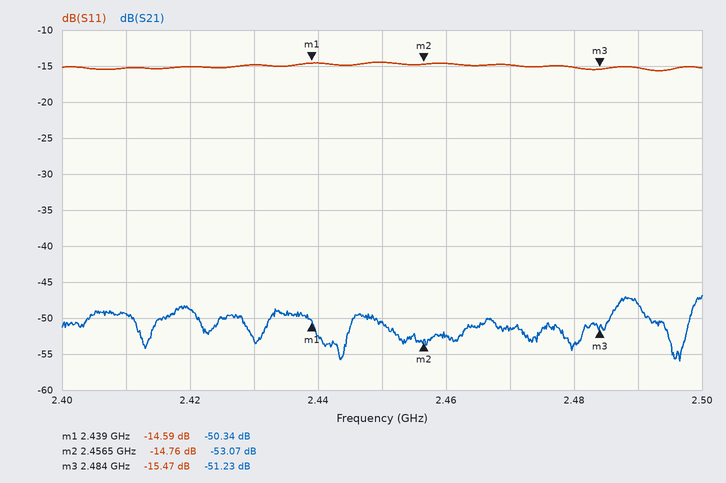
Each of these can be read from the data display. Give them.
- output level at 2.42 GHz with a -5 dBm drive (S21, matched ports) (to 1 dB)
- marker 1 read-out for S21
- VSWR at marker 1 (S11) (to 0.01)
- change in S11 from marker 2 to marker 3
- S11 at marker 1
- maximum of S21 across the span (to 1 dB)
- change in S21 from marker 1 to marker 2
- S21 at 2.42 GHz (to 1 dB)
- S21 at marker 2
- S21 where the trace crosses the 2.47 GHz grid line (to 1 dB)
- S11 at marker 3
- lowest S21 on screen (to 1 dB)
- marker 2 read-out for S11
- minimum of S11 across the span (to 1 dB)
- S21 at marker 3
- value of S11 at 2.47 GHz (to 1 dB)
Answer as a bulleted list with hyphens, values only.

- -54 dBm
- -50.34 dB
- 1.46
- -0.71 dB
- -14.59 dB
- -47 dB
- -2.73 dB
- -49 dB
- -53.07 dB
- -51 dB
- -15.47 dB
- -56 dB
- -14.76 dB
- -16 dB
- -51.23 dB
- -15 dB
